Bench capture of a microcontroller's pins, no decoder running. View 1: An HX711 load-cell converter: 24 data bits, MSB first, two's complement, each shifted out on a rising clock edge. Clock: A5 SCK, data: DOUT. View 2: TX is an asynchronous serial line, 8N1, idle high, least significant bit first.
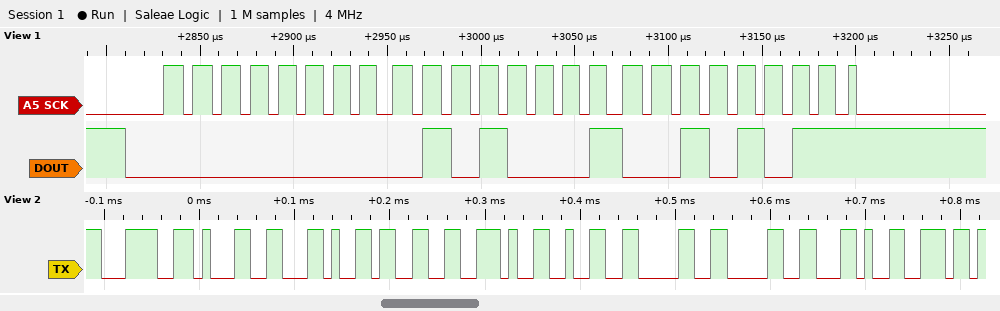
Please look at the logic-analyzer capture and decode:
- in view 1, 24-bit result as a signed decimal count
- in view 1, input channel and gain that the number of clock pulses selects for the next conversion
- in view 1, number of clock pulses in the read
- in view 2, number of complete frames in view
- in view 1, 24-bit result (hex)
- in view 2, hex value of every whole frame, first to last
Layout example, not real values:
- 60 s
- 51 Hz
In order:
- 20779
- channel A, gain 128
- 25
- 10
- 0x00512B
- 3C 31 2C 33 2E 32 30 30 2C 6E
